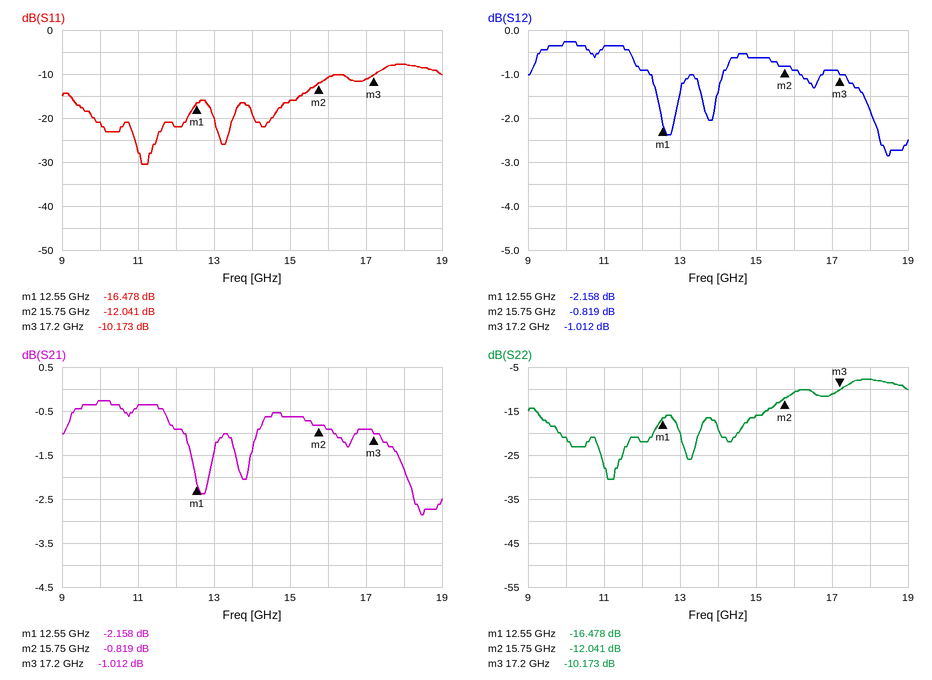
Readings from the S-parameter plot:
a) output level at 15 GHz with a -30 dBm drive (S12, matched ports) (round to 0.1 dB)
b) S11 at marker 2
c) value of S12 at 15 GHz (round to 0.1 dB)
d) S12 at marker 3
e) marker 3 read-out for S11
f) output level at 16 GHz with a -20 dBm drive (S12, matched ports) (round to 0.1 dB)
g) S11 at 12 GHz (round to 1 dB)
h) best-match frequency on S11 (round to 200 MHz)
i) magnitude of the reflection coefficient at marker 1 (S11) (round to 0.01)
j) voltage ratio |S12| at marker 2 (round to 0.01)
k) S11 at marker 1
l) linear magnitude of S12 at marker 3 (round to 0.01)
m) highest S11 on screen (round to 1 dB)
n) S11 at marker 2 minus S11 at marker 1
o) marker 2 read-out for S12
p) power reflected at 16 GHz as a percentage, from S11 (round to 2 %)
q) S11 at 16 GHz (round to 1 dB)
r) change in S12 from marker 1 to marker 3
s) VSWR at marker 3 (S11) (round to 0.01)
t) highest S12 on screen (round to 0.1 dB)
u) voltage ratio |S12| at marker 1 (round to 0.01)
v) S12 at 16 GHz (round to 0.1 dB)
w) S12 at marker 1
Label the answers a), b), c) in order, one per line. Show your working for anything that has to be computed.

a) -30 dBm + (-0.6 dB) = -30.6 dBm
b) -12.041 dB
c) -0.6 dB
d) -1.012 dB
e) -10.173 dB
f) -20 dBm + (-0.9 dB) = -20.9 dBm
g) -22 dB
h) 11.2 GHz
i) 10^(-16.478/20) ≈ 0.15
j) 10^(-0.819/20) ≈ 0.91
k) -16.478 dB
l) 10^(-1.012/20) ≈ 0.89
m) -8 dB
n) -12.041 − (-16.478) = 4.437 dB
o) -0.819 dB
p) 10^(-11/10) ≈ 8 %
q) -11 dB
r) -1.012 − (-2.158) = 1.146 dB
s) (1 + 0.3100)/(1 − 0.3100) ≈ 1.90
t) -0.3 dB
u) 10^(-2.158/20) ≈ 0.78
v) -0.9 dB
w) -2.158 dB
